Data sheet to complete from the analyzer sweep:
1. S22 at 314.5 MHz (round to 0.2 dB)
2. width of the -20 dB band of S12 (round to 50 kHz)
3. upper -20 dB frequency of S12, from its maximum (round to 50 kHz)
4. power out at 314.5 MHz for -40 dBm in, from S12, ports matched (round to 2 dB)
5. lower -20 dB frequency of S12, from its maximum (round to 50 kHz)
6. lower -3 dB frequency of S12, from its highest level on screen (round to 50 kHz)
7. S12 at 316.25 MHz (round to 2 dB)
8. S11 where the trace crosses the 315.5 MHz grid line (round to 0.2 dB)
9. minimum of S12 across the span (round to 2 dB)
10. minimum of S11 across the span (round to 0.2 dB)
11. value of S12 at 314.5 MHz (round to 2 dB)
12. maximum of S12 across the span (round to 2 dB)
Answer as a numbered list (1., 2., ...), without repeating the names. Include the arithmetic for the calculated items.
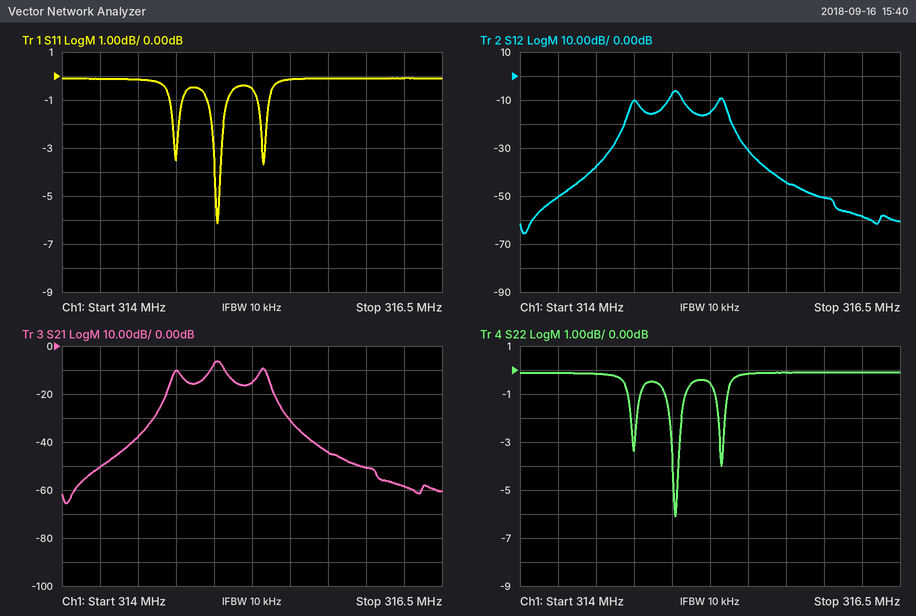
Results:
1. -0.2 dB
2. 315.45 MHz − 314.65 MHz = 800 kHz
3. 315.45 MHz
4. -40 dBm + (-38 dB) = -78 dBm
5. 314.65 MHz
6. 315.00 MHz
7. -58 dB
8. -0.2 dB
9. -66 dB
10. -6.2 dB
11. -38 dB
12. -6 dB
